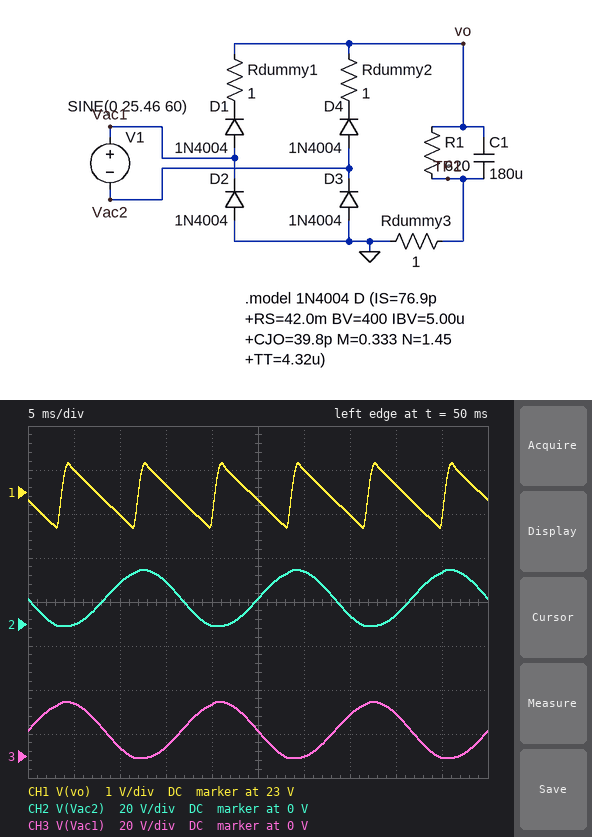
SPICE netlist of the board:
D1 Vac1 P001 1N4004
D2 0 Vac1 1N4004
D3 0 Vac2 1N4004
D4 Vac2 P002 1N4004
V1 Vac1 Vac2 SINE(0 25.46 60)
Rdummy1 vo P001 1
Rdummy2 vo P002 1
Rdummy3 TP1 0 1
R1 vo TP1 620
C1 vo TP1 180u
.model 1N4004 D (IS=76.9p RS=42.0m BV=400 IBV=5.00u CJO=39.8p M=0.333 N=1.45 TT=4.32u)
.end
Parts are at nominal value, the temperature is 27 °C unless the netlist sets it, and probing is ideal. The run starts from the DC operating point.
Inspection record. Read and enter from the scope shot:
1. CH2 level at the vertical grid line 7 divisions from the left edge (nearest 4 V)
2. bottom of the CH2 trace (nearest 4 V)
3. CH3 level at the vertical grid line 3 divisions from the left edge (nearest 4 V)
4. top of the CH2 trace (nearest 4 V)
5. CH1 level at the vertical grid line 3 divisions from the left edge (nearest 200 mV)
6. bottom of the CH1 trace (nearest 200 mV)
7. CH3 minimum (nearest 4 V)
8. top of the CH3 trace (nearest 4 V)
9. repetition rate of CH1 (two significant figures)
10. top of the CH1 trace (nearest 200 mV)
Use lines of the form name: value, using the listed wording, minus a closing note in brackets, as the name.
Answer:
CH2 level at the vertical grid line 7 divisions from the left edge: 4 V
bottom of the CH2 trace: 0 V
CH3 level at the vertical grid line 3 divisions from the left edge: 4 V
top of the CH2 trace: 24 V
CH1 level at the vertical grid line 3 divisions from the left edge: 23.2 V
bottom of the CH1 trace: 22.2 V
CH3 minimum: 0 V
top of the CH3 trace: 24 V
repetition rate of CH1: 120 Hz
top of the CH1 trace: 23.6 V
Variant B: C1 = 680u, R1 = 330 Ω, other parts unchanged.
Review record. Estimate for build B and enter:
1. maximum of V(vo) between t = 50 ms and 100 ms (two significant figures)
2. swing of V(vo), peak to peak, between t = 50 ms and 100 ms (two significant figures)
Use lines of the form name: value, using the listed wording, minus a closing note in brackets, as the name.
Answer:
maximum of V(vo) between t = 50 ms and 100 ms: 23 V
swing of V(vo), peak to peak, between t = 50 ms and 100 ms: 960 mV
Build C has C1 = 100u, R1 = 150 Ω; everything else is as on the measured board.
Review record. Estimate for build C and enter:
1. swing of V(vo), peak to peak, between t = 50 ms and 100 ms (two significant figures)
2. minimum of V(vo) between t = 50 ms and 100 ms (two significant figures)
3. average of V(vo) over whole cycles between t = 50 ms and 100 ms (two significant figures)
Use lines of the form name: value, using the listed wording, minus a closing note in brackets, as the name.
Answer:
swing of V(vo), peak to peak, between t = 50 ms and 100 ms: 7.5 V
minimum of V(vo) between t = 50 ms and 100 ms: 16 V
average of V(vo) over whole cycles between t = 50 ms and 100 ms: 20 V
